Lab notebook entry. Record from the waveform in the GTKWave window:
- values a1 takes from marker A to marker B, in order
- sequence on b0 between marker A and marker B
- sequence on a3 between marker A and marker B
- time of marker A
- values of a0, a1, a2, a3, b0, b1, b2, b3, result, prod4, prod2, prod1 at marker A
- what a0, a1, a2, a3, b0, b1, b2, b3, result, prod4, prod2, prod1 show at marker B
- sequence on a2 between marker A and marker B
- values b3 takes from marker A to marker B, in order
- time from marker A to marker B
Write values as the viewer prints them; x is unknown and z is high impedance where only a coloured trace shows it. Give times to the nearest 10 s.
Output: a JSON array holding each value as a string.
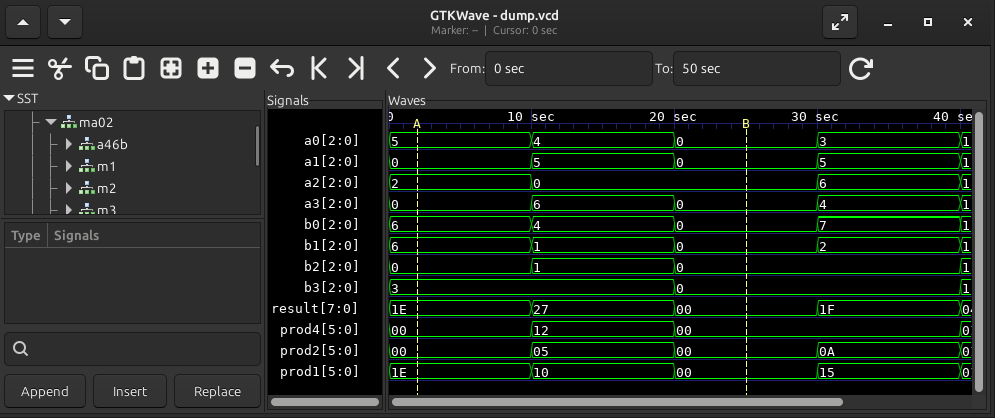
["0, 5, 0", "6, 4, 0", "0, 6, 0", "0 s", "a0=5, a1=0, a2=2, a3=0, b0=6, b1=6, b2=0, b3=3, result=1E, prod4=00, prod2=00, prod1=1E", "a0=0, a1=0, a2=0, a3=0, b0=0, b1=0, b2=0, b3=0, result=00, prod4=00, prod2=00, prod1=00", "2, 0", "3, 0", "20 s"]
